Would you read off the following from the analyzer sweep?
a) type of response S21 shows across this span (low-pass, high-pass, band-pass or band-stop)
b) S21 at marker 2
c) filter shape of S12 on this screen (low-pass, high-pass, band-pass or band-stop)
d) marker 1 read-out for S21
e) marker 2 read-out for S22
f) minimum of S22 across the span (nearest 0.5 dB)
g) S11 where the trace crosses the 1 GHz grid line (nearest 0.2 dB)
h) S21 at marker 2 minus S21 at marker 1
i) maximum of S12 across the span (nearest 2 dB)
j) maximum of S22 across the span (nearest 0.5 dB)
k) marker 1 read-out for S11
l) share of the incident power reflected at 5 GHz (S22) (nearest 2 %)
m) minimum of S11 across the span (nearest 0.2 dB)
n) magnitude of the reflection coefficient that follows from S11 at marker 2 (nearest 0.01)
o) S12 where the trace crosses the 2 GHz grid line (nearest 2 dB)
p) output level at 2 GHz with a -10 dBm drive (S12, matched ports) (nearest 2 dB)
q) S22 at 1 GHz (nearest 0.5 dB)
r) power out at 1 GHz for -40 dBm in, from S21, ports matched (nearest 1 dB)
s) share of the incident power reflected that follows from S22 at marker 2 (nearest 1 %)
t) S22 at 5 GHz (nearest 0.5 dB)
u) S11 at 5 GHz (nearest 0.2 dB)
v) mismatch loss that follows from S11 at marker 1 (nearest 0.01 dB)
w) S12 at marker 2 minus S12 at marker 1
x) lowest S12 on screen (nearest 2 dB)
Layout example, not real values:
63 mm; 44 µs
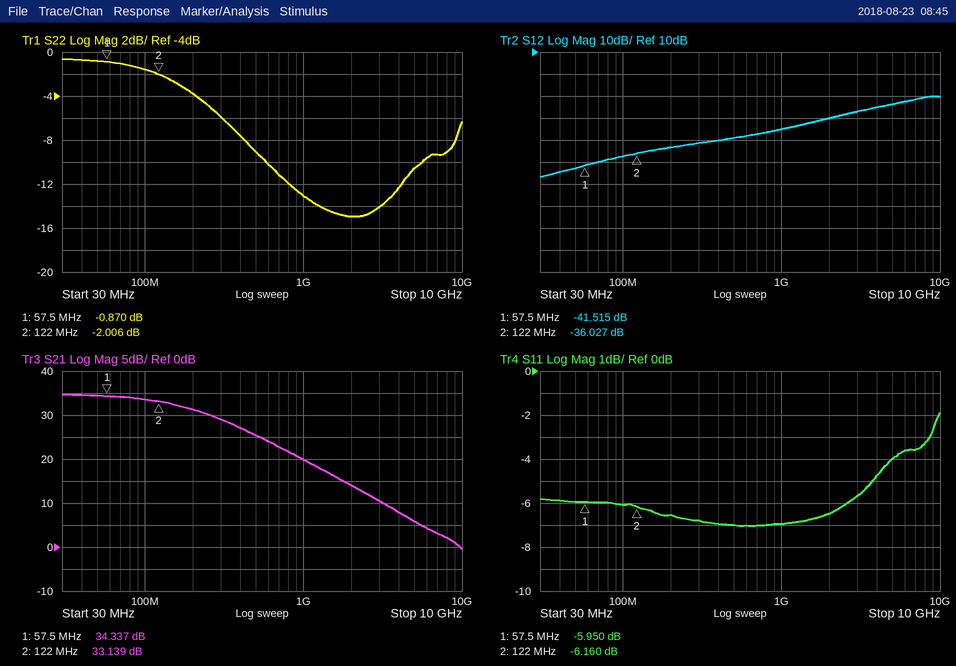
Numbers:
low-pass; 33.139 dB; high-pass; 34.337 dB; -2.006 dB; -15.0 dB; -7.0 dB; -1.198 dB; -10 dB; -0.5 dB; -5.950 dB; 8 %; -7.0 dB; 0.49; -20 dB; -30 dBm; -13.0 dB; -20 dBm; 63 %; -10.5 dB; -4.0 dB; 1.27 dB; 5.488 dB; -46 dB
